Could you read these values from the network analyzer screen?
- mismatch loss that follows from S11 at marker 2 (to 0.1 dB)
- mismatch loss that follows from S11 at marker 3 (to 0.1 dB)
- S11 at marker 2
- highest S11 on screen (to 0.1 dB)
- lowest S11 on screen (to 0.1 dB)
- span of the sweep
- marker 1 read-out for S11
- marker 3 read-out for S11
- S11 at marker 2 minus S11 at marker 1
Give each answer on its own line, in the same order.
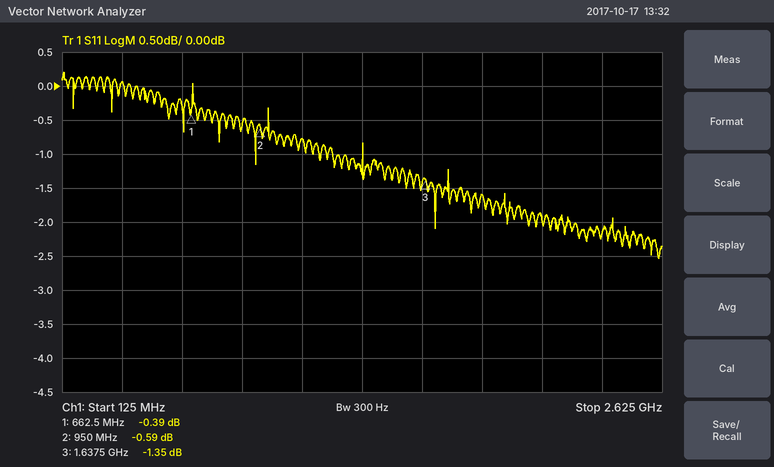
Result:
9.0 dB
5.7 dB
-0.59 dB
0.2 dB
-2.5 dB
2.5 GHz
-0.39 dB
-1.35 dB
-0.20 dB
